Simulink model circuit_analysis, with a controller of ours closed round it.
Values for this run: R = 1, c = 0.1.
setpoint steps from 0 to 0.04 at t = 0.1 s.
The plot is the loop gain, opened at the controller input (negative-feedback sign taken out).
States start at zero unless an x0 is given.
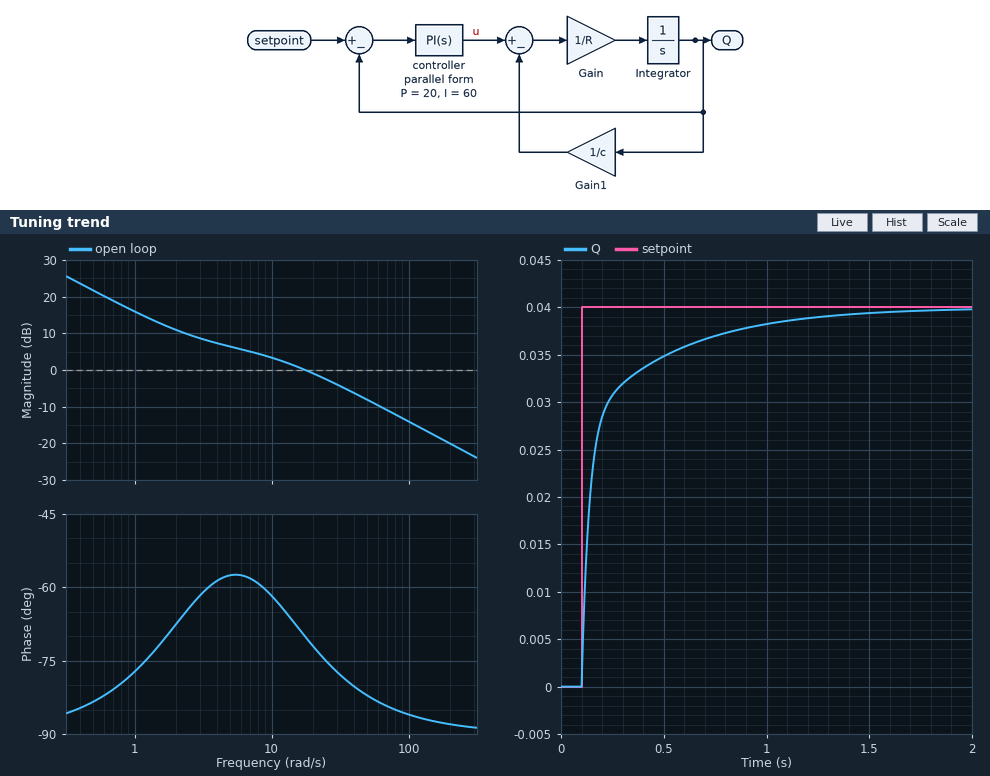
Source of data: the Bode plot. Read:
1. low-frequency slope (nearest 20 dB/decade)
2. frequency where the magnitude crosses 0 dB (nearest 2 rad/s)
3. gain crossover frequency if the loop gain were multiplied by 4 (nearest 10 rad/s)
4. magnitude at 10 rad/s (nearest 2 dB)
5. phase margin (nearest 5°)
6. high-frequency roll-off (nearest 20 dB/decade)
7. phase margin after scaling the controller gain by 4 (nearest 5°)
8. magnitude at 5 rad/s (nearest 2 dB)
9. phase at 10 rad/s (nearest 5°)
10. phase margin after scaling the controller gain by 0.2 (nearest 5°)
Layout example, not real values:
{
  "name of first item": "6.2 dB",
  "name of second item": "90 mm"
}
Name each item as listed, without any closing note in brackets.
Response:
{
  "low-frequency slope": "-20 dB/decade",
  "frequency where the magnitude crosses 0 dB": "18 rad/s",
  "gain crossover frequency if the loop gain were multiplied by 4": "80 rad/s",
  "magnitude at 10 rad/s": "4 dB",
  "phase margin": "110°",
  "high-frequency roll-off": "-20 dB/decade",
  "phase margin after scaling the controller gain by 4": "95°",
  "magnitude at 5 rad/s": "6 dB",
  "phase at 10 rad/s": "-60°",
  "phase margin after scaling the controller gain by 0.2": "105°"
}
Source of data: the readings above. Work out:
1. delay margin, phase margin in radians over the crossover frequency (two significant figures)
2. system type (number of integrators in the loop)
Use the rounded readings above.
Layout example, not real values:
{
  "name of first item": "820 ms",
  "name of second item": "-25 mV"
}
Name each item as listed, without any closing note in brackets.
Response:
{
  "delay margin, phase margin in radians over the crossover frequency": "0.11 s",
  "system type": "1"
}
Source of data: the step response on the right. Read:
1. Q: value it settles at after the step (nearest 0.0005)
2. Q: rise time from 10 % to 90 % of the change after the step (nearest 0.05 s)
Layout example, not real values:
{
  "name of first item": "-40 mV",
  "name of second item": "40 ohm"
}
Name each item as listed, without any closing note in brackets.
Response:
{
  "Q: value it settles at after the step": "0.0400",
  "Q: rise time from 10 % to 90 % of the change after the step": "0.50 s"
}
